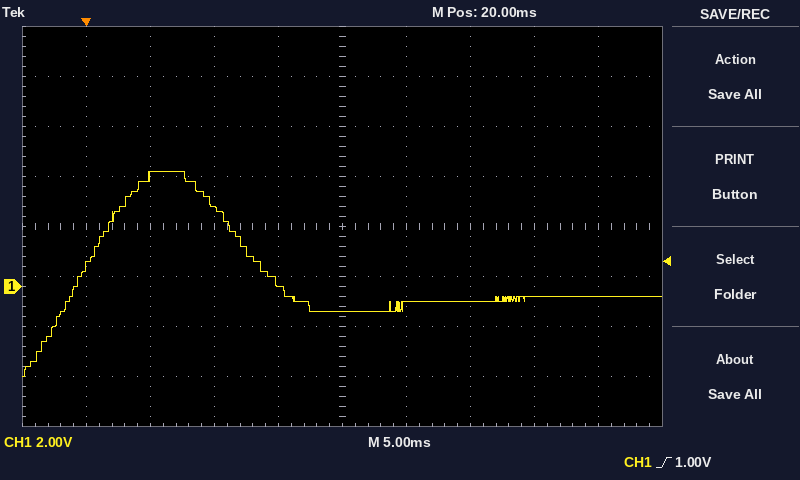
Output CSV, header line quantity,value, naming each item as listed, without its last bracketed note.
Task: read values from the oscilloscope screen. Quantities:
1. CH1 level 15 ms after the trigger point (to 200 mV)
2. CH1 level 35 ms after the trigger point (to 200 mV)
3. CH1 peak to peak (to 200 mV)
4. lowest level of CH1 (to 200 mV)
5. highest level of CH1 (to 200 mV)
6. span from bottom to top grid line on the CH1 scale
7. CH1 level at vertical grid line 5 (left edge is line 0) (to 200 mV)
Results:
quantity,value
CH1 level 15 ms after the trigger point,200 mV
CH1 level 35 ms after the trigger point,-400 mV
CH1 peak to peak,8.2 V
lowest level of CH1,-3.6 V
highest level of CH1,4.6 V
span from bottom to top grid line on the CH1 scale,16 V
CH1 level at vertical grid line 5 (left edge is line 0),-1.0 V
